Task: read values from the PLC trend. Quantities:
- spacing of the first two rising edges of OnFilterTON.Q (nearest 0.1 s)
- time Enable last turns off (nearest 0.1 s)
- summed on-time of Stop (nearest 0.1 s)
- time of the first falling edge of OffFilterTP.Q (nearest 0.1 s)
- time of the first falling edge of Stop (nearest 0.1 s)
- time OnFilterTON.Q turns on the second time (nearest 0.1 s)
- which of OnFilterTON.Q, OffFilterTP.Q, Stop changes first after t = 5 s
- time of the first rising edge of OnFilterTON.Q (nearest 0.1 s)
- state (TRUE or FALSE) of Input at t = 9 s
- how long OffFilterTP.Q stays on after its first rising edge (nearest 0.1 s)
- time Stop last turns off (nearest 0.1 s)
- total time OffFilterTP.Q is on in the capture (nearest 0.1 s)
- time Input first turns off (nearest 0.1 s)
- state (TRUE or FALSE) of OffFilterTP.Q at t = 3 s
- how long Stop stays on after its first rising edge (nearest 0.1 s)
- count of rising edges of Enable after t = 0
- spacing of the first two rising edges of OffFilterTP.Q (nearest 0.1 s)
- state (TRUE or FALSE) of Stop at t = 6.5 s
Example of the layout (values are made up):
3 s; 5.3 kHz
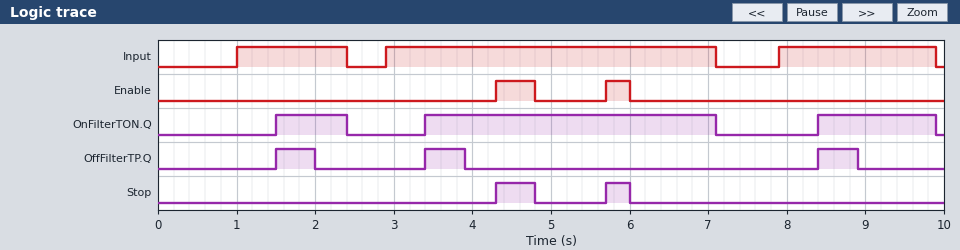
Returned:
1.9 s; 6.0 s; 0.8 s; 2.0 s; 4.8 s; 3.4 s; Stop; 1.5 s; TRUE; 0.5 s; 6.0 s; 1.5 s; 2.4 s; FALSE; 0.5 s; 2; 1.9 s; FALSE
